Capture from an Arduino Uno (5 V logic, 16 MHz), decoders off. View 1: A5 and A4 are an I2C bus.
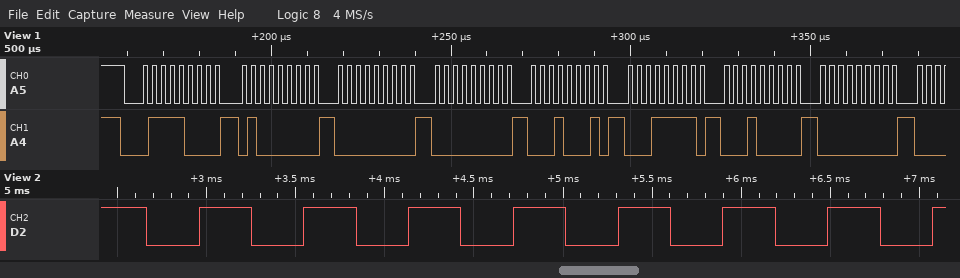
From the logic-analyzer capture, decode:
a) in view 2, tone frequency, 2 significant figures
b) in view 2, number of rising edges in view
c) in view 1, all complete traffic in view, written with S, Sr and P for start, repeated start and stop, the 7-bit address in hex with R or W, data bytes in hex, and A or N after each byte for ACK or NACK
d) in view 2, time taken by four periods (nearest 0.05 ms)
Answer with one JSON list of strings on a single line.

["1.7 kHz", "8", "S 3CW A 40 A 00 A 00 A 11 A 1F A 10 A 00 A", "2.35 ms"]
